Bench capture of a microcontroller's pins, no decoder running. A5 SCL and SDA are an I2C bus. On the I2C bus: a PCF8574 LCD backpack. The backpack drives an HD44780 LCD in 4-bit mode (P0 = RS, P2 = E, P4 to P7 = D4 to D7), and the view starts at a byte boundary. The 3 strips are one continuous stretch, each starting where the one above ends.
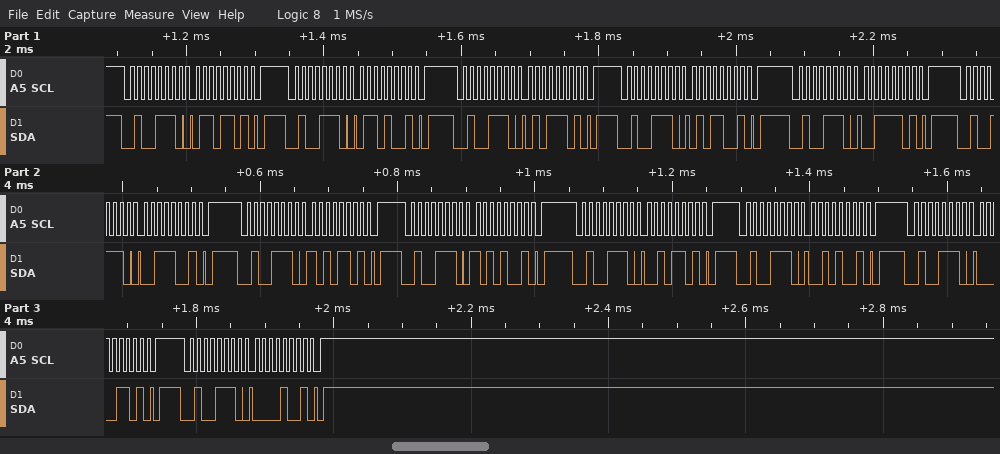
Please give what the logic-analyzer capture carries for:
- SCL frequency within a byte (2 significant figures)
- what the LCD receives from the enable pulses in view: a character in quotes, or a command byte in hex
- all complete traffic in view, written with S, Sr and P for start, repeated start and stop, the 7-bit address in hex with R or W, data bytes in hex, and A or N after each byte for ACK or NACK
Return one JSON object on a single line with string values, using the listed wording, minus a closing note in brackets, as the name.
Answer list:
{"SCL frequency within a byte": "100 kHz", "what the LCD receives from the enable pulses in view: a character in quotes, or a command byte in hex": "'e' ':' ' '", "all complete traffic in view, written with S, Sr and P for start, repeated start and stop, the 7-bit address in hex with R or W, data bytes in hex, and A or N after each byte for ACK or NACK": "S 27W A 6D A P S 27W A 69 A P S 27W A 5D A P S 27W A 59 A P S 27W A 3D A P S 27W A 39 A P S 27W A AD A P S 27W A A9 A P S 27W A 2D A P S 27W A 29 A P S 27W A 0D A P S 27W A 09 A P"}
